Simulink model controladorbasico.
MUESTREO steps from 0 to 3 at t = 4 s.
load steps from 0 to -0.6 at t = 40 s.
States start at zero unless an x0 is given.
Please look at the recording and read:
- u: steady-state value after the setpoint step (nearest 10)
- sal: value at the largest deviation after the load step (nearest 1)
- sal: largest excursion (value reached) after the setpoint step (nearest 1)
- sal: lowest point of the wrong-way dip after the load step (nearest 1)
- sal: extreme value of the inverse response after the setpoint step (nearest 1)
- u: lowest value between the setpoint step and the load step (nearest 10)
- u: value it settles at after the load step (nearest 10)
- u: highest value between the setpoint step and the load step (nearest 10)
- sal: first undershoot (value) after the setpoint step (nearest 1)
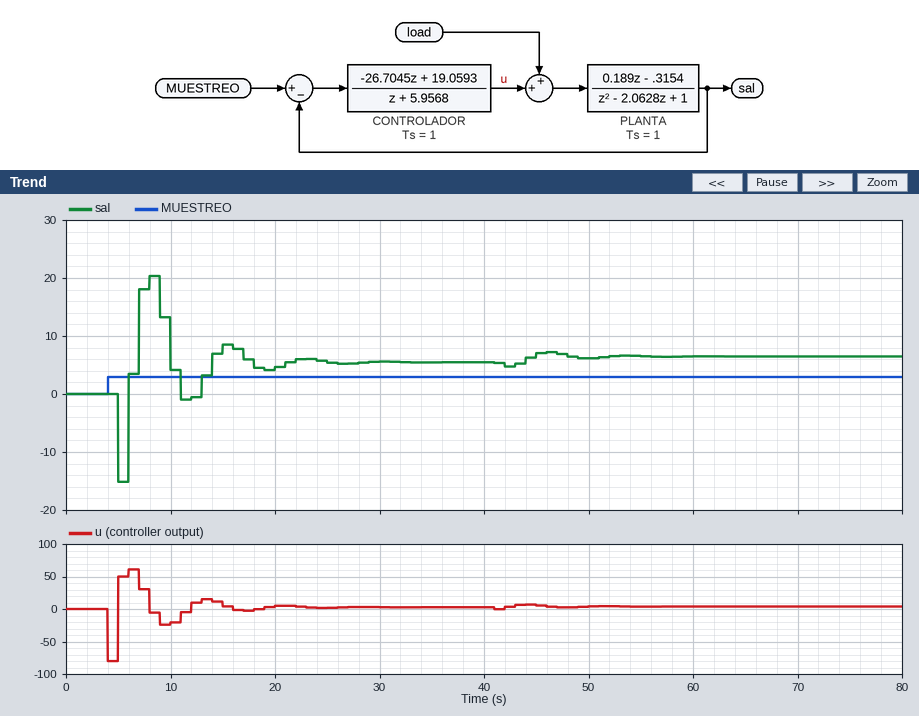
0
7
20
5
-15
-80
0
60
-1
